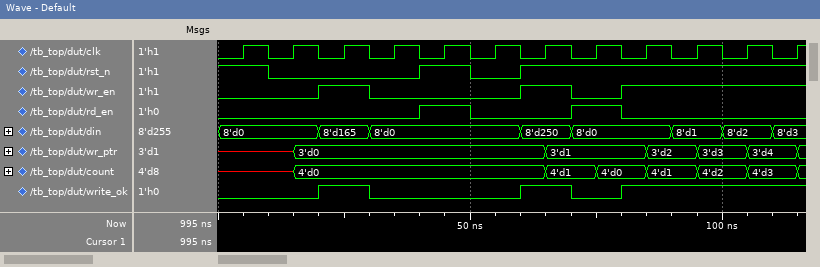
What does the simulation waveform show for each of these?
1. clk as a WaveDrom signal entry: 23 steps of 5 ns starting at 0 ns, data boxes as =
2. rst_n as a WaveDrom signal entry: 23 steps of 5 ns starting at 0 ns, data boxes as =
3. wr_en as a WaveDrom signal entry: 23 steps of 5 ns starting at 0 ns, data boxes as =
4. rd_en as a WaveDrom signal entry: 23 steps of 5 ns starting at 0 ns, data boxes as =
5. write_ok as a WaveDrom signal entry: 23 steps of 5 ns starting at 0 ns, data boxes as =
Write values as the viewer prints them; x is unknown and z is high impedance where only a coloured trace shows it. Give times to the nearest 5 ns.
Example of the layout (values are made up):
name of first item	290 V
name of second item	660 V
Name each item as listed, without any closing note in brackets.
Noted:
clk as a WaveDrom signal entry: 23 steps of 5 ns starting at 0 ns, data boxes as =	{name: 'clk', wave: '01010101010101010101010'}
rst_n as a WaveDrom signal entry: 23 steps of 5 ns starting at 0 ns, data boxes as =	{name: 'rst_n', wave: '1.0.....1.0.1..........'}
wr_en as a WaveDrom signal entry: 23 steps of 5 ns starting at 0 ns, data boxes as =	{name: 'wr_en', wave: '0...1.0.....1.0.1......'}
rd_en as a WaveDrom signal entry: 23 steps of 5 ns starting at 0 ns, data boxes as =	{name: 'rd_en', wave: '0.......1.0...1.0......'}
write_ok as a WaveDrom signal entry: 23 steps of 5 ns starting at 0 ns, data boxes as =	{name: 'write_ok', wave: '0...1.0.....1.0.1......'}
